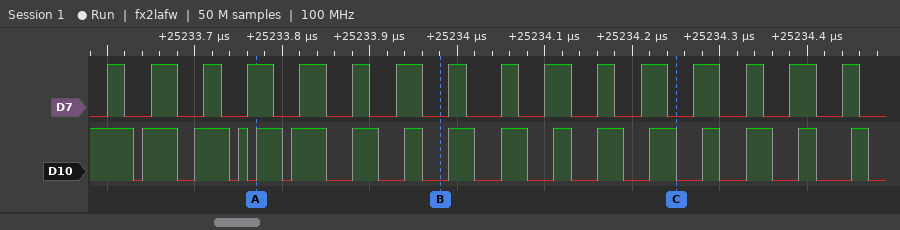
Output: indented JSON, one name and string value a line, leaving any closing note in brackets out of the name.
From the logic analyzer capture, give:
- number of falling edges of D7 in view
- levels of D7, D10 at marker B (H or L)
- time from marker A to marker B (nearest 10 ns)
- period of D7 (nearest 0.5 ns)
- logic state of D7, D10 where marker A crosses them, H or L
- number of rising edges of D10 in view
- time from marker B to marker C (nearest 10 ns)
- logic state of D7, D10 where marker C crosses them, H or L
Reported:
{
  "number of falling edges of D7 in view": "16",
  "levels of D7, D10 at marker B": "D7=L, D10=L",
  "time from marker A to marker B": "210 ns",
  "period of D7": "56 ns",
  "logic state of D7, D10 where marker A crosses them, H or L": "D7=H, D10=H",
  "number of rising edges of D10 in view": "16",
  "time from marker B to marker C": "270 ns",
  "logic state of D7, D10 where marker C crosses them, H or L": "D7=L, D10=L"
}
